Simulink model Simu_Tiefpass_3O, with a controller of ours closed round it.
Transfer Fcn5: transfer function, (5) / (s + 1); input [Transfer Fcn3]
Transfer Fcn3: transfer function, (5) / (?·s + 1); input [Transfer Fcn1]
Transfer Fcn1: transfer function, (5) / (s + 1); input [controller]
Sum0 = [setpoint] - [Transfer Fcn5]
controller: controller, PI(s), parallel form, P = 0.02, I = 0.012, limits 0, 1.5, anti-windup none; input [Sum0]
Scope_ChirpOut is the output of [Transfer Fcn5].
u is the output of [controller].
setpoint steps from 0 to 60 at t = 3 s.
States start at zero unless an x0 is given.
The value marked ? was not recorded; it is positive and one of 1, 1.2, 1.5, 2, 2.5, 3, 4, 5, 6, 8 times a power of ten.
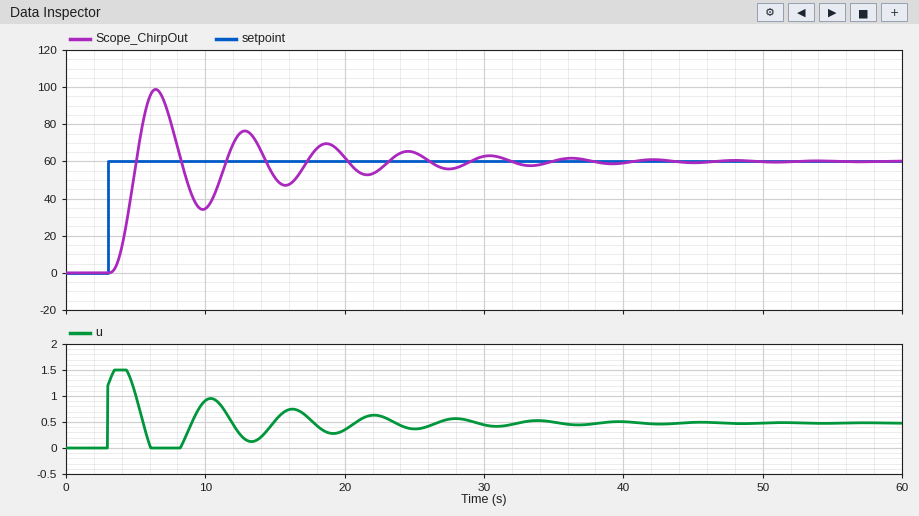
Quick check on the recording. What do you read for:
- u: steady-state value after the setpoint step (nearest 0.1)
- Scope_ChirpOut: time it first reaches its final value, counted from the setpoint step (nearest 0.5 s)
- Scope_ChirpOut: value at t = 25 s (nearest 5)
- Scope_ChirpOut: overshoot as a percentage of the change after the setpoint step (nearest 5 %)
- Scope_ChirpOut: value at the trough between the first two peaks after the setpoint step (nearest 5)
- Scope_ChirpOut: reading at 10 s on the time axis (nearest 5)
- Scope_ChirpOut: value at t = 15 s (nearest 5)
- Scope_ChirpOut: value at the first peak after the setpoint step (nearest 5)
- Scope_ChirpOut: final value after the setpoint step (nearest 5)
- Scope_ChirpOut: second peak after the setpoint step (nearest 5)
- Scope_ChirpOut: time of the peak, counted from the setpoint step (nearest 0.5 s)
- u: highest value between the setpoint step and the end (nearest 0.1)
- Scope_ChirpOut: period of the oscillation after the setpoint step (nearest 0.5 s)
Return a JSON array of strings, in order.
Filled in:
["0.5", "2.0 s", "65", "65 %", "35", "35", "50", "100", "60", "75", "3.5 s", "1.5", "6.5 s"]
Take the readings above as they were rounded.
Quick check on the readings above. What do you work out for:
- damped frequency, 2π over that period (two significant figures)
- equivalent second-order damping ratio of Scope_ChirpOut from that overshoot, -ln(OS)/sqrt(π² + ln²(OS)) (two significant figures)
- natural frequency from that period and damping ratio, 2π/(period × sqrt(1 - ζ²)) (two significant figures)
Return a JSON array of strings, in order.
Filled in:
["0.97 rad/s", "0.14", "0.98 rad/s"]
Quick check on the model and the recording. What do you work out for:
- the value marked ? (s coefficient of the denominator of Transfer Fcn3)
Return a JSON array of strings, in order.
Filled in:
["1"]
